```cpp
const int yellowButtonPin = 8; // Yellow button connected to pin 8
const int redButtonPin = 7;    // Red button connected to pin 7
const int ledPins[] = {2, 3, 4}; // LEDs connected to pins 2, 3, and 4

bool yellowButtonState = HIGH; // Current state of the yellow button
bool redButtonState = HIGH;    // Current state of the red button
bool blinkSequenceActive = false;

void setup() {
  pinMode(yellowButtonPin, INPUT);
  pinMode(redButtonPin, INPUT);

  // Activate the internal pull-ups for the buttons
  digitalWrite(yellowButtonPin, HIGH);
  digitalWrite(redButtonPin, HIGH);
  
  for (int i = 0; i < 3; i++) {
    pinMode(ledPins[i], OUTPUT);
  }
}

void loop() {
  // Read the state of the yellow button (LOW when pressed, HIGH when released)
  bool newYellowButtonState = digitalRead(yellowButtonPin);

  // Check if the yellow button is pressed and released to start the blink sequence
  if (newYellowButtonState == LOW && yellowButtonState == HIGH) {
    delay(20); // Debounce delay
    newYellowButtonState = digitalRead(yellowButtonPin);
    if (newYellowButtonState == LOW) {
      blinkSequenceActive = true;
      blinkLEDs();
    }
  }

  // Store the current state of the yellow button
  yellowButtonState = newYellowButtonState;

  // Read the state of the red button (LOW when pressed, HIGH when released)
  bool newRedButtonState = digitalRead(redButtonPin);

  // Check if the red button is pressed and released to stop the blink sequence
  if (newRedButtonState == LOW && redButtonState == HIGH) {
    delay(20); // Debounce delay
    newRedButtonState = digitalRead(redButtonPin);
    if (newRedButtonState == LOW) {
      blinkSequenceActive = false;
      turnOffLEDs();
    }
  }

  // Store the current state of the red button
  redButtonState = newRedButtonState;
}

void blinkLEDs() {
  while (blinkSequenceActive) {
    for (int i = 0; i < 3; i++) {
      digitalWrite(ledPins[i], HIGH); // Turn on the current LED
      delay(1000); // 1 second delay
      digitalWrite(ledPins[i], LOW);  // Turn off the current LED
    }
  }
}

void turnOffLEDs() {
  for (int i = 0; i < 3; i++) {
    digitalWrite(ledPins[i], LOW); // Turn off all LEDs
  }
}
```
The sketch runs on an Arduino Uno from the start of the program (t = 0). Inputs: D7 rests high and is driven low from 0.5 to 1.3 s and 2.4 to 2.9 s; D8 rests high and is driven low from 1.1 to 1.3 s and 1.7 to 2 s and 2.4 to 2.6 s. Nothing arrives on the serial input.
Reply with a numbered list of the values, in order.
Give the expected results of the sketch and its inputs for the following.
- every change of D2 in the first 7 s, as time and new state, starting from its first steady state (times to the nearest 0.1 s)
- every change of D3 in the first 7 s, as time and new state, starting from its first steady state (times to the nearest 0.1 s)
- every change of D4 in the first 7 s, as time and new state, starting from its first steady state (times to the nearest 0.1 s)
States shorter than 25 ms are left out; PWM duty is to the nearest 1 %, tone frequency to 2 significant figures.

1. 0 s low; 1.1 s high; 2.1 s low; 4.1 s high; 5.1 s low
2. 0 s low; 2.1 s high; 3.1 s low; 5.1 s high; 6.1 s low
3. 0 s low; 3.1 s high; 4.1 s low; 6.1 s high
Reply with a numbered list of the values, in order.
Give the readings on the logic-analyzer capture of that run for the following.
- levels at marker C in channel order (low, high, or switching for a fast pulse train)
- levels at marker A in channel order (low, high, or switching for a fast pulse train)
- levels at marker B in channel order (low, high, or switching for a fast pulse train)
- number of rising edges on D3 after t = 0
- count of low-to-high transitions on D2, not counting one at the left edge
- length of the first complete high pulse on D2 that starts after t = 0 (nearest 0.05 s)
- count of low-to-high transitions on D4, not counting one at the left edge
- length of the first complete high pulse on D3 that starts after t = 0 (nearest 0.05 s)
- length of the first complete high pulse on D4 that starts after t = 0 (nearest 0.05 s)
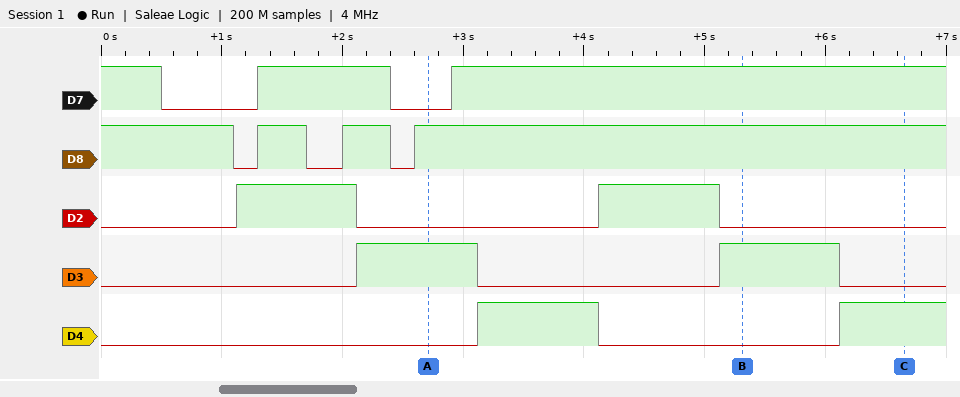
1. D7 high, D8 high, D2 low, D3 low, D4 high
2. D7 low, D8 high, D2 low, D3 high, D4 low
3. D7 high, D8 high, D2 low, D3 high, D4 low
4. 2
5. 2
6. 1.00 s
7. 2
8. 1.00 s
9. 1.00 s
